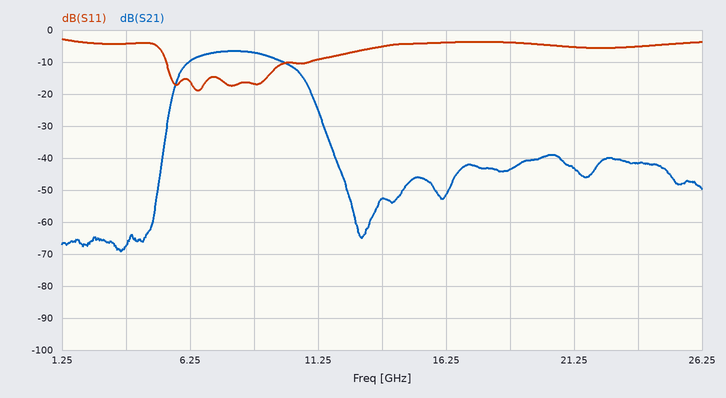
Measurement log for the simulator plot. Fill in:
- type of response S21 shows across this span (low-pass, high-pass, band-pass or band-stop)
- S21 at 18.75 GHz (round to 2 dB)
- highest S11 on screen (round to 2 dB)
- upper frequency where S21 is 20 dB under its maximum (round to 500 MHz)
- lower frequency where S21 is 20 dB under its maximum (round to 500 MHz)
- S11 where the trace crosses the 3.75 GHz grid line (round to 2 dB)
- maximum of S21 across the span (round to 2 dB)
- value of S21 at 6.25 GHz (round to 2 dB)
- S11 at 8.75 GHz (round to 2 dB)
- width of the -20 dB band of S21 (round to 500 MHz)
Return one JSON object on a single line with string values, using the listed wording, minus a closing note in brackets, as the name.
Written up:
{"type of response S21 shows across this span": "band-pass", "S21 at 18.75 GHz": "-44 dB", "highest S11 on screen": "-2 dB", "upper frequency where S21 is 20 dB under its maximum": "11.5 GHz", "lower frequency where S21 is 20 dB under its maximum": "5.5 GHz", "S11 where the trace crosses the 3.75 GHz grid line": "-4 dB", "maximum of S21 across the span": "-6 dB", "value of S21 at 6.25 GHz": "-10 dB", "S11 at 8.75 GHz": "-16 dB", "width of the -20 dB band of S21": "6.0 GHz"}
